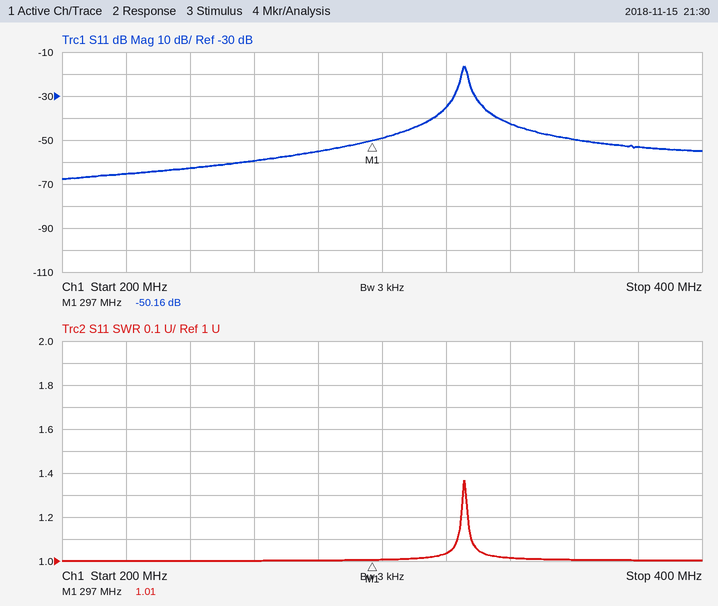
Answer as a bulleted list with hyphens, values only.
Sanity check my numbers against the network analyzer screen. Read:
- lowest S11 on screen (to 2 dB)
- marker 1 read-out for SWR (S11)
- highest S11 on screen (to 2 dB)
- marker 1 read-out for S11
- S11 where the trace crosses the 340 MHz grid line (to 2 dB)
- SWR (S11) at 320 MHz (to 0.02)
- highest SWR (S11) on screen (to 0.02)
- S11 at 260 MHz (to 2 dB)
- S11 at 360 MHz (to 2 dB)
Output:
- -68 dB
- 1.01
- -16 dB
- -50.16 dB
- -42 dB
- 1.04
- 1.36
- -60 dB
- -50 dB
